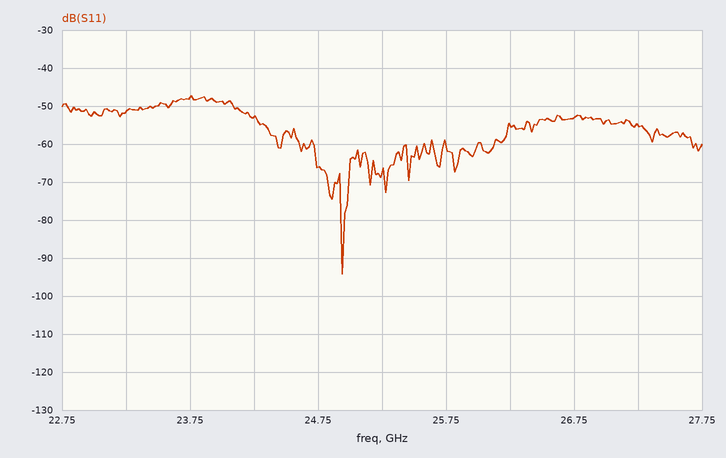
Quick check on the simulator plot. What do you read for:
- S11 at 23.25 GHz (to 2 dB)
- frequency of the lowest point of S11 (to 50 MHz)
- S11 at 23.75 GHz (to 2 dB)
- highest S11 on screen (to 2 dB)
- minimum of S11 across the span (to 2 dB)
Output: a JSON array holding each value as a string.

["-52 dB", "24.95 GHz", "-48 dB", "-48 dB", "-94 dB"]
